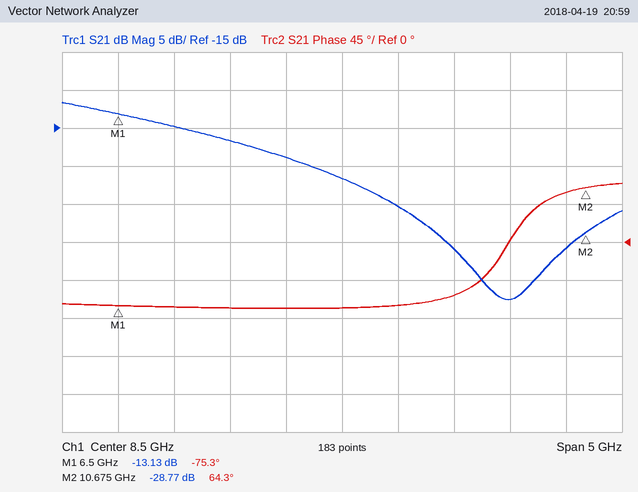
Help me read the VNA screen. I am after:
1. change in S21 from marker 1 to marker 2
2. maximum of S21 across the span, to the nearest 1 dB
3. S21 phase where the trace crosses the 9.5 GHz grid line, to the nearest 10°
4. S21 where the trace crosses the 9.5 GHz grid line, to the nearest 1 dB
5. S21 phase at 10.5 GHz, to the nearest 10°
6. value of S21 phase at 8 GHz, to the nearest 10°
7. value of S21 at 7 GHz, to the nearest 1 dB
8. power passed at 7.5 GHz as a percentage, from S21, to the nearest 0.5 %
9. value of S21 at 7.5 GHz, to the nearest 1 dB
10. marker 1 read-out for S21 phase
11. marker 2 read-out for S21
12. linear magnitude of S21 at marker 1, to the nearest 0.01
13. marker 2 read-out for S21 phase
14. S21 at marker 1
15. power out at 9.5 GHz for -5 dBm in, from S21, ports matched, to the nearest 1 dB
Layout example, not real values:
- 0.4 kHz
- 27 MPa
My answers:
- -15.64 dB
- -12 dB
- -60°
- -31 dB
- 60°
- -80°
- -15 dB
- 2.0 %
- -17 dB
- -75.3°
- -28.77 dB
- 0.22
- 64.3°
- -13.13 dB
- -36 dBm
